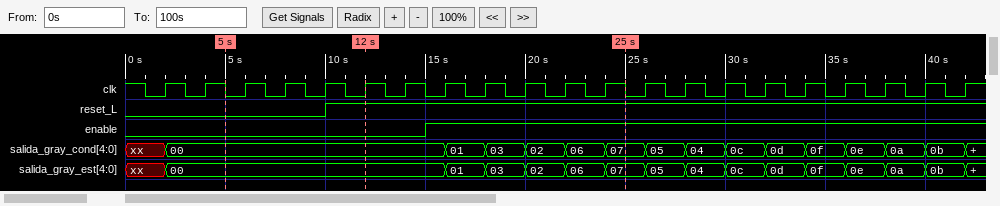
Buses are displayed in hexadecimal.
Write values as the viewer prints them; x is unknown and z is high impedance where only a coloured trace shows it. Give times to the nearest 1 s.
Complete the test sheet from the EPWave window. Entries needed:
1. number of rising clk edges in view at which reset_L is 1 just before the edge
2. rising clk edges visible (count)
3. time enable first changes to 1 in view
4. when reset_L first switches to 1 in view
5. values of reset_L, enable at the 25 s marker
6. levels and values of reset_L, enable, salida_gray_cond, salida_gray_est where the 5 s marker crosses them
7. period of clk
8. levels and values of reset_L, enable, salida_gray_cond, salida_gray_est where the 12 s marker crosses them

16
21
15 s
10 s
reset_L=1, enable=1
reset_L=0, enable=0, salida_gray_cond=00, salida_gray_est=00
2 s
reset_L=1, enable=0, salida_gray_cond=00, salida_gray_est=00
